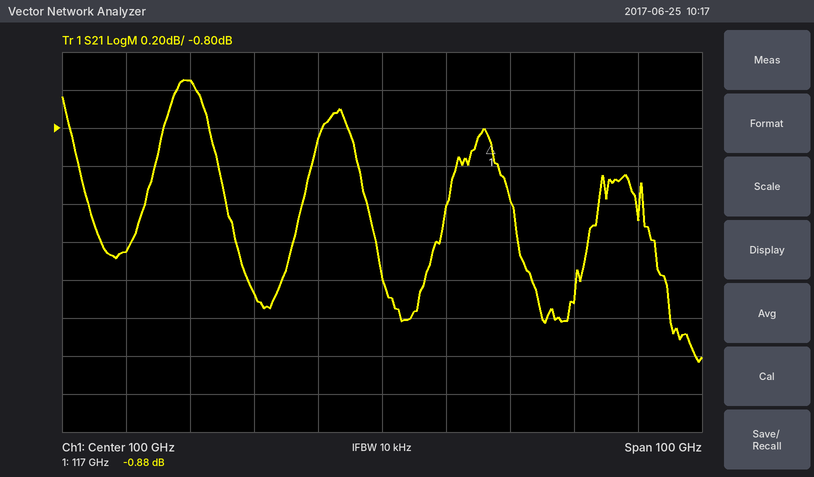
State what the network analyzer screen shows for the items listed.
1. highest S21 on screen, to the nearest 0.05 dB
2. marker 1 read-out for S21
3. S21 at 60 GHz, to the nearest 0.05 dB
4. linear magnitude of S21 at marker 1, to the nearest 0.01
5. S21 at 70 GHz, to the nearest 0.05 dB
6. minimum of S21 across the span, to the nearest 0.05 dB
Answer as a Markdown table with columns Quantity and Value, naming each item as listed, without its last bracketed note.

| Quantity | Value |
|---|---|
| highest S21 on screen, to the nearest 0.05 dB | -0.55 dB |
| marker 1 read-out for S21 | -0.88 dB |
| S21 at 60 GHz, to the nearest 0.05 dB | -1.45 dB |
| linear magnitude of S21 at marker 1, to the nearest 0.01 | 0.90 |
| S21 at 70 GHz, to the nearest 0.05 dB | -0.55 dB |
| minimum of S21 across the span, to the nearest 0.05 dB | -2.05 dB |
